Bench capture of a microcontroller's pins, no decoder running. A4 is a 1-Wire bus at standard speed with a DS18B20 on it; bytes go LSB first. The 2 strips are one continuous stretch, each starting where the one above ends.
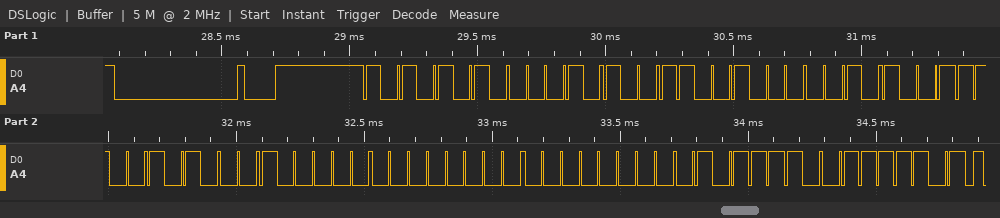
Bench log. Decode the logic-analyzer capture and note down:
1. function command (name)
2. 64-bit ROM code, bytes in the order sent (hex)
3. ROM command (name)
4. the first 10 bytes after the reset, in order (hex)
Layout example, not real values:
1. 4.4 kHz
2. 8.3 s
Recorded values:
1. Read Scratchpad
2. 28 13 94 53 04 00 00 7A
3. Match ROM
4. 55 28 13 94 53 04 00 00 7A BE
